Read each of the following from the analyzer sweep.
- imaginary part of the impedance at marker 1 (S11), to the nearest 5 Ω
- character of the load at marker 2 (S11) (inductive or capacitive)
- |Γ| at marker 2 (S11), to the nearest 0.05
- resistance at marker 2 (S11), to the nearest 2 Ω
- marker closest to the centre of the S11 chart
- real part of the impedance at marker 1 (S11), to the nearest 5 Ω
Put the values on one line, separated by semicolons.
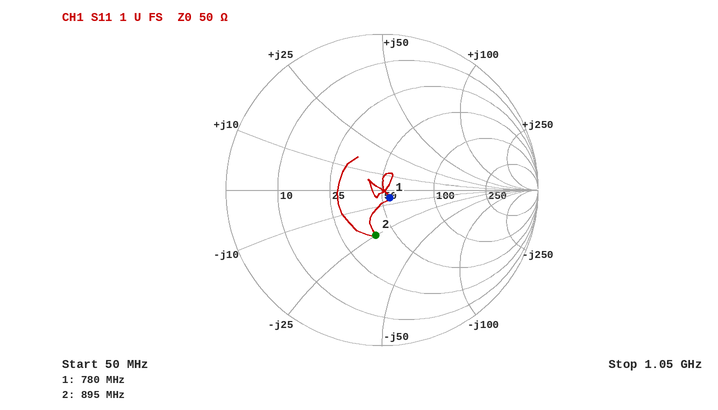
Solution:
-5 Ω; capacitive; 0.30; 40 Ω; marker 1; 55 Ω
